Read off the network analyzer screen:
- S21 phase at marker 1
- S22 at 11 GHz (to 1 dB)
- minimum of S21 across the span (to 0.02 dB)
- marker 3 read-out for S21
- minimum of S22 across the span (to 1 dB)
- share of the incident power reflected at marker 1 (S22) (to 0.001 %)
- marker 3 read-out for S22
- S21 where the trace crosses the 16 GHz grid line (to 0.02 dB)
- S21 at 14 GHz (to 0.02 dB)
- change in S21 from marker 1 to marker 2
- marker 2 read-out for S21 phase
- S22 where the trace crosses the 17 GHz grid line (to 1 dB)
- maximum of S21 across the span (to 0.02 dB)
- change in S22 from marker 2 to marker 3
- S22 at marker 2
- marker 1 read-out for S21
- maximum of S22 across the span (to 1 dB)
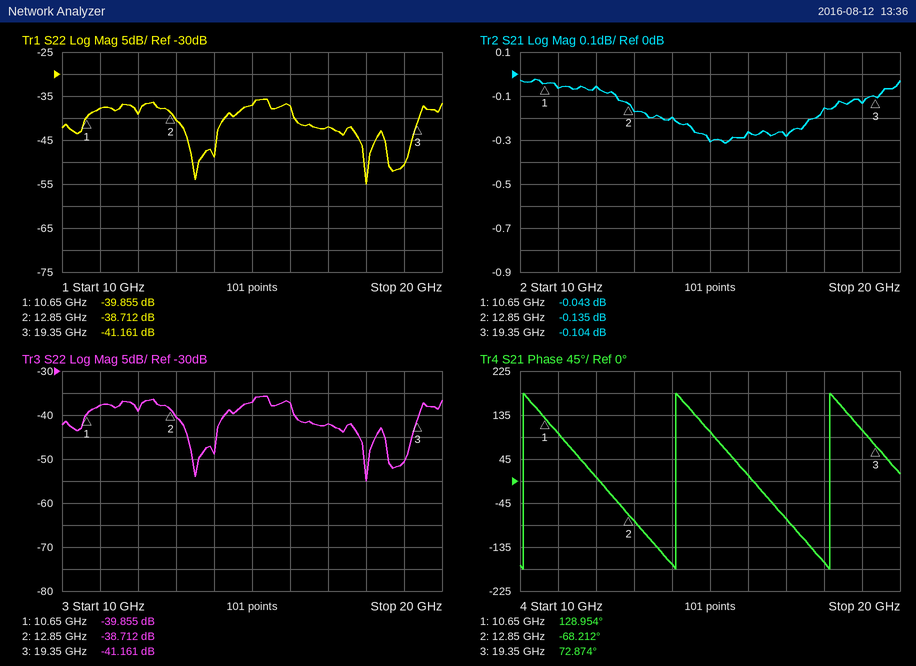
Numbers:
128.954°
-38 dB
-0.32 dB
-0.104 dB
-55 dB
0.010 %
-41.161 dB
-0.26 dB
-0.20 dB
-0.092 dB
-68.212°
-42 dB
-0.02 dB
-2.449 dB
-38.712 dB
-0.043 dB
-36 dB
